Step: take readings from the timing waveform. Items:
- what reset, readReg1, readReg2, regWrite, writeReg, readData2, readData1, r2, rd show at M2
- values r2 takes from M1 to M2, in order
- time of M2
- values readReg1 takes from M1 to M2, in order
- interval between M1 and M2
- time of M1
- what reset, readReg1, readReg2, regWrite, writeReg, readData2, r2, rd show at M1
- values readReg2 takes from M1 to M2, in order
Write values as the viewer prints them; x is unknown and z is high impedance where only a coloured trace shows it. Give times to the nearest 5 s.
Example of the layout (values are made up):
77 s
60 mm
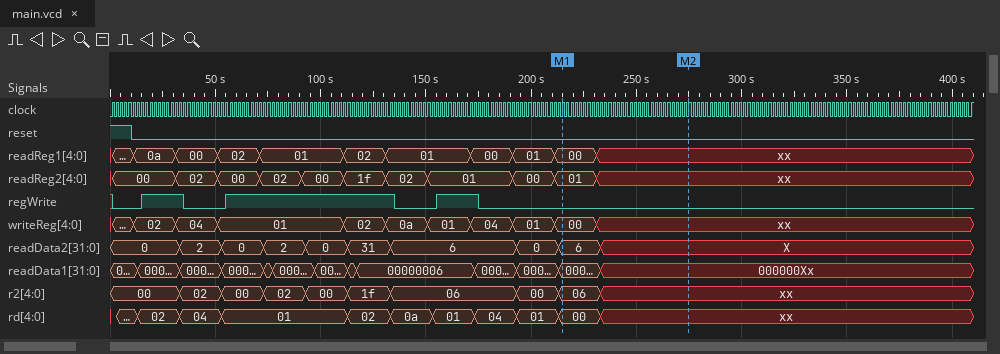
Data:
reset=0, readReg1=xx, readReg2=xx, regWrite=0, writeReg=xx, readData2=X, readData1=000000Xx, r2=xx, rd=xx
06, xx
275 s
00, xx
60 s
215 s
reset=0, readReg1=00, readReg2=01, regWrite=0, writeReg=00, readData2=6, r2=06, rd=00
01, xx
